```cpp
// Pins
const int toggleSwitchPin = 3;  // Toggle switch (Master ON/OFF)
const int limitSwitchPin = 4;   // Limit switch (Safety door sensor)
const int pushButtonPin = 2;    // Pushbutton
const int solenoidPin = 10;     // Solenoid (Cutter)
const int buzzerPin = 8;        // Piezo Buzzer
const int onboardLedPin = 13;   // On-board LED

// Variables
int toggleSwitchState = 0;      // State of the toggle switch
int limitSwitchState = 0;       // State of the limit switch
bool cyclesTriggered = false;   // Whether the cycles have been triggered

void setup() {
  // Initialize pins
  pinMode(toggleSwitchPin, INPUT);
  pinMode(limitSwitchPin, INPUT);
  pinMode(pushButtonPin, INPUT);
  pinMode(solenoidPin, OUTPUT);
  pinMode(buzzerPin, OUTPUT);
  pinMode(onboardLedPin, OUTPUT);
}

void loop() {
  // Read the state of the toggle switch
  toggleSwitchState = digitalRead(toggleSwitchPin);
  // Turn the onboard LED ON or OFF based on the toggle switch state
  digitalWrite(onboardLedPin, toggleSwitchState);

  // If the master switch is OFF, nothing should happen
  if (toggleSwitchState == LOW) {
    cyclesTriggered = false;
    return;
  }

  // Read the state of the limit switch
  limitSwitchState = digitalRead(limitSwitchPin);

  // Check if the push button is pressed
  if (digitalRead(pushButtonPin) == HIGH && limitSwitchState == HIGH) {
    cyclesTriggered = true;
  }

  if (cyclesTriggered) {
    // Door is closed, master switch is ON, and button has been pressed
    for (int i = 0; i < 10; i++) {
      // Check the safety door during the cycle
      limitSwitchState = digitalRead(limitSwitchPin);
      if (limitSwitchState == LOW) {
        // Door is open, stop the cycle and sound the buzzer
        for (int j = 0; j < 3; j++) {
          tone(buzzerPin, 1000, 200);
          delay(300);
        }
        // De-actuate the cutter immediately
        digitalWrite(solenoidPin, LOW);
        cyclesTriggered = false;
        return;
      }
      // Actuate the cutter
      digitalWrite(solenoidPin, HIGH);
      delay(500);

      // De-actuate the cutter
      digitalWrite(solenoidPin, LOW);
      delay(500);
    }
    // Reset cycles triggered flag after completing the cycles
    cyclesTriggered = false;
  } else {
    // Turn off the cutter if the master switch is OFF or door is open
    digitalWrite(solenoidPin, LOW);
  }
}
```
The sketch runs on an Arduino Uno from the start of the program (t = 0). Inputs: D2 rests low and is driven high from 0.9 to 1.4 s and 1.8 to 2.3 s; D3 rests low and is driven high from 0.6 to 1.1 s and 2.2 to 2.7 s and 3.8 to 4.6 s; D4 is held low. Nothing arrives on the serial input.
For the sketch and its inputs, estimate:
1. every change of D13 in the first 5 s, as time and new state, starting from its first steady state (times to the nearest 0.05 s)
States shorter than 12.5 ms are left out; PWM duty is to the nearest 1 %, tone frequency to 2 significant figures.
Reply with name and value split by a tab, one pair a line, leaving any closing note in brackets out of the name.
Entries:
every change of D13 in the first 5 s, as time and new state, starting from its first steady state	0 s low; 0.6 s high; 1.1 s low; 2.2 s high; 2.7 s low; 3.8 s high; 4.6 s low
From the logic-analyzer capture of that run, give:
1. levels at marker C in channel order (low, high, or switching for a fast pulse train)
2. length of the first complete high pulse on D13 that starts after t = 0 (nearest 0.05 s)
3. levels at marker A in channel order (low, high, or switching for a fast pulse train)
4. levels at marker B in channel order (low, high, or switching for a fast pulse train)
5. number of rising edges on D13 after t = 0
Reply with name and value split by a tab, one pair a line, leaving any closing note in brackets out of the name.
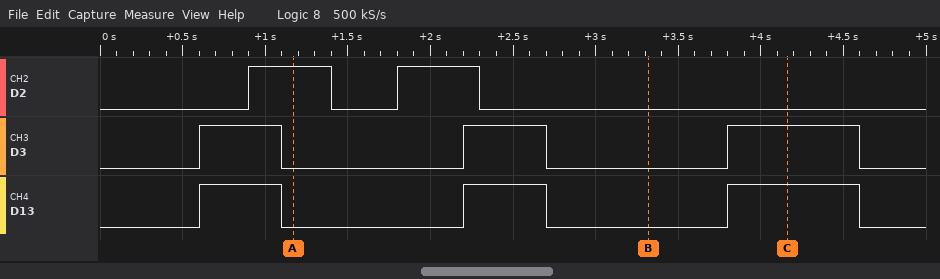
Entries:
levels at marker C in channel order	D2 low, D3 high, D13 high
length of the first complete high pulse on D13 that starts after t = 0	0.50 s
levels at marker A in channel order	D2 high, D3 low, D13 low
levels at marker B in channel order	D2 low, D3 low, D13 low
number of rising edges on D13 after t = 0	3
